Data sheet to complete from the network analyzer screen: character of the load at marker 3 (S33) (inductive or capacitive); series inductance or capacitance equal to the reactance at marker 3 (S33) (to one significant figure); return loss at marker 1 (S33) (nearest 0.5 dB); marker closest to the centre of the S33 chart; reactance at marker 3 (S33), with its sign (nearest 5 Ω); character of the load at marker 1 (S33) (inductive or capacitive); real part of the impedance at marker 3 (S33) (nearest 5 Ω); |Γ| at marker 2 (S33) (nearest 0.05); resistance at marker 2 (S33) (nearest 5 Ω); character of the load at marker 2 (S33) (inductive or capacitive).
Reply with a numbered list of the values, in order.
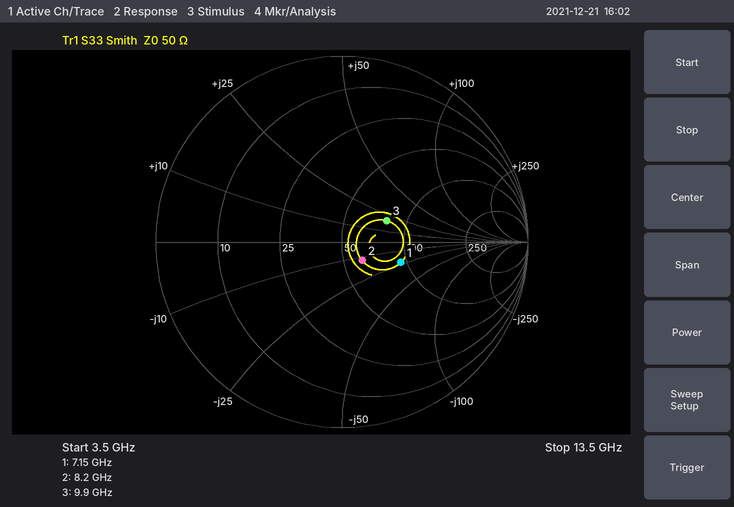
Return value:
1. inductive
2. 300 pH
3. 9.5 dB
4. marker 2
5. +20 Ω
6. capacitive
7. 80 Ω
8. 0.15
9. 60 Ω
10. capacitive
